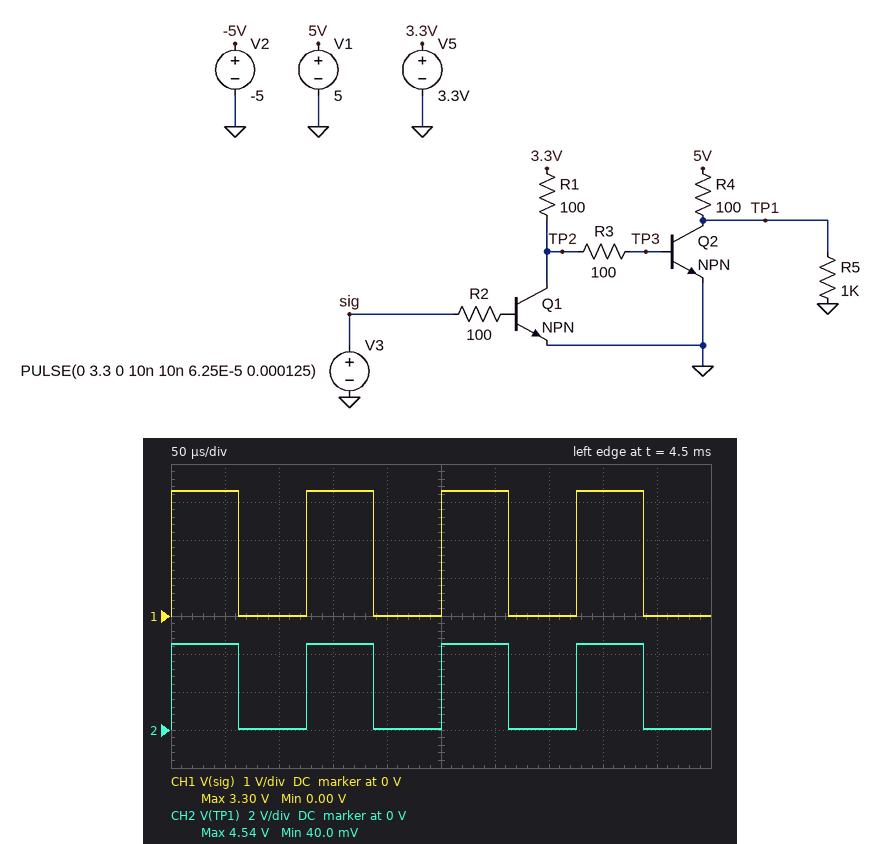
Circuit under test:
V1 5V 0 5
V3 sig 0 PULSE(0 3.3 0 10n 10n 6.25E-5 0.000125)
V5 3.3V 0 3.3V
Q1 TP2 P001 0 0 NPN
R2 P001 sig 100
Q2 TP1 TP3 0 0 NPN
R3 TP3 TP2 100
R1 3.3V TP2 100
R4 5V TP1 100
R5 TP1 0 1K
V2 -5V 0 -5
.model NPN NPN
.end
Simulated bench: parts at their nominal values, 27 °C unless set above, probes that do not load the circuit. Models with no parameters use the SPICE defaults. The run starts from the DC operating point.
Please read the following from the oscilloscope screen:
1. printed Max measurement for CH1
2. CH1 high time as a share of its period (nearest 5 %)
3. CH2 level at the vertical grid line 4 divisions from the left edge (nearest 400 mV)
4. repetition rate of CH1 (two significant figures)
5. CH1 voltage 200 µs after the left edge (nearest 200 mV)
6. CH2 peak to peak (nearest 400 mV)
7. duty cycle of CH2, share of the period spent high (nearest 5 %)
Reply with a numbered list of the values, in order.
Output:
1. 3.30 V
2. 50 %
3. 0 V
4. 8.0 kHz
5. 0 V
6. 4.4 V
7. 50 %
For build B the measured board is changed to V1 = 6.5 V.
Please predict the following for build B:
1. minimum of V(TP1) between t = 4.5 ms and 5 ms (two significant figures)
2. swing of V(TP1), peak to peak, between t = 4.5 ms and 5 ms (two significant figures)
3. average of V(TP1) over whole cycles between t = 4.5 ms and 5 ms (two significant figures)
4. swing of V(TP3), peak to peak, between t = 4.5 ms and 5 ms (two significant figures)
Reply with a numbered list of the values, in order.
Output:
1. 53 mV
2. 5.9 V
3. 3.0 V
4. 860 mV
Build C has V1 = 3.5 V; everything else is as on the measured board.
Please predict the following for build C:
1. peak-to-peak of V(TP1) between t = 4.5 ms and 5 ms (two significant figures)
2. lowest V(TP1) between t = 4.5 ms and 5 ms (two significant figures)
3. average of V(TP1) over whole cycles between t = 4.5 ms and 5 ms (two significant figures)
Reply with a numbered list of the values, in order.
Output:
1. 3.1 V
2. 42 mV
3. 1.6 V
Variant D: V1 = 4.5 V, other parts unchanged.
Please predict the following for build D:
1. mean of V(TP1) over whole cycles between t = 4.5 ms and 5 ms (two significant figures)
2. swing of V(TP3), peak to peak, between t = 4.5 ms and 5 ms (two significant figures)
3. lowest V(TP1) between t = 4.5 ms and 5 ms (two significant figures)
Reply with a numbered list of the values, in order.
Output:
1. 2.1 V
2. 850 mV
3. 46 mV
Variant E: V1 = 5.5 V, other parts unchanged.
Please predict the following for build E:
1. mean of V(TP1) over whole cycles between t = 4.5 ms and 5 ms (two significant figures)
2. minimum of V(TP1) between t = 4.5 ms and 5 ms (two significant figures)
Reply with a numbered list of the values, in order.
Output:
1. 2.5 V
2. 50 mV
